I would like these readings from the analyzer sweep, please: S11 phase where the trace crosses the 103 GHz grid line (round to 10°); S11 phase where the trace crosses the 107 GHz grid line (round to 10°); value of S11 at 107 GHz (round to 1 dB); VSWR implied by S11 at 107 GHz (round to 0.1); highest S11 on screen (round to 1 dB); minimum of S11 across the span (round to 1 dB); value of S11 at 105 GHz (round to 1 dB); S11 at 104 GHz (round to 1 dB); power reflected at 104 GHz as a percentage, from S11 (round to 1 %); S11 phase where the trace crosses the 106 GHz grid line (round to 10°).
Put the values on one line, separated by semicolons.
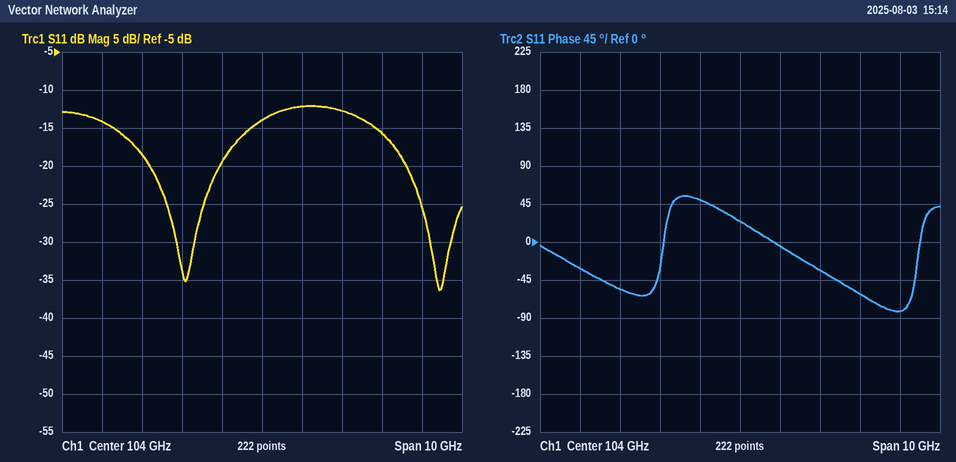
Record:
50°; -60°; -16 dB; 1.4; -12 dB; -36 dB; -12 dB; -14 dB; 4 %; -30°
